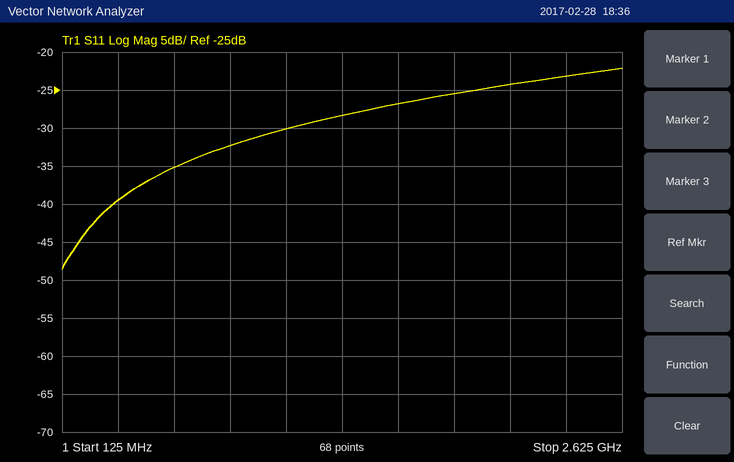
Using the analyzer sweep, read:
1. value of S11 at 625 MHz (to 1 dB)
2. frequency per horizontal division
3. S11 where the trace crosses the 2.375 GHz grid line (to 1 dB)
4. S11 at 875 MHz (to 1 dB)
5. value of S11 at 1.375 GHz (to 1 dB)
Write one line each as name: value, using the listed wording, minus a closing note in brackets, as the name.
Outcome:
value of S11 at 625 MHz: -35 dB
frequency per horizontal division: 250 MHz
S11 where the trace crosses the 2.375 GHz grid line: -23 dB
S11 at 875 MHz: -32 dB
value of S11 at 1.375 GHz: -28 dB
